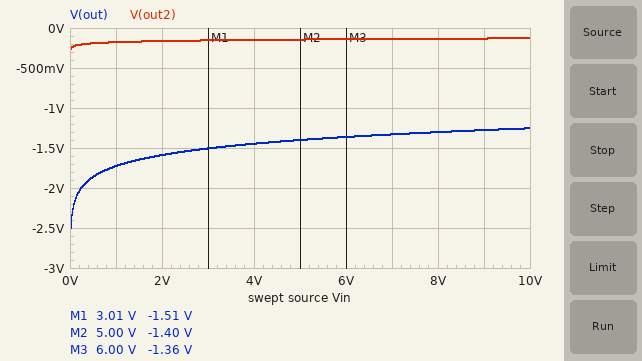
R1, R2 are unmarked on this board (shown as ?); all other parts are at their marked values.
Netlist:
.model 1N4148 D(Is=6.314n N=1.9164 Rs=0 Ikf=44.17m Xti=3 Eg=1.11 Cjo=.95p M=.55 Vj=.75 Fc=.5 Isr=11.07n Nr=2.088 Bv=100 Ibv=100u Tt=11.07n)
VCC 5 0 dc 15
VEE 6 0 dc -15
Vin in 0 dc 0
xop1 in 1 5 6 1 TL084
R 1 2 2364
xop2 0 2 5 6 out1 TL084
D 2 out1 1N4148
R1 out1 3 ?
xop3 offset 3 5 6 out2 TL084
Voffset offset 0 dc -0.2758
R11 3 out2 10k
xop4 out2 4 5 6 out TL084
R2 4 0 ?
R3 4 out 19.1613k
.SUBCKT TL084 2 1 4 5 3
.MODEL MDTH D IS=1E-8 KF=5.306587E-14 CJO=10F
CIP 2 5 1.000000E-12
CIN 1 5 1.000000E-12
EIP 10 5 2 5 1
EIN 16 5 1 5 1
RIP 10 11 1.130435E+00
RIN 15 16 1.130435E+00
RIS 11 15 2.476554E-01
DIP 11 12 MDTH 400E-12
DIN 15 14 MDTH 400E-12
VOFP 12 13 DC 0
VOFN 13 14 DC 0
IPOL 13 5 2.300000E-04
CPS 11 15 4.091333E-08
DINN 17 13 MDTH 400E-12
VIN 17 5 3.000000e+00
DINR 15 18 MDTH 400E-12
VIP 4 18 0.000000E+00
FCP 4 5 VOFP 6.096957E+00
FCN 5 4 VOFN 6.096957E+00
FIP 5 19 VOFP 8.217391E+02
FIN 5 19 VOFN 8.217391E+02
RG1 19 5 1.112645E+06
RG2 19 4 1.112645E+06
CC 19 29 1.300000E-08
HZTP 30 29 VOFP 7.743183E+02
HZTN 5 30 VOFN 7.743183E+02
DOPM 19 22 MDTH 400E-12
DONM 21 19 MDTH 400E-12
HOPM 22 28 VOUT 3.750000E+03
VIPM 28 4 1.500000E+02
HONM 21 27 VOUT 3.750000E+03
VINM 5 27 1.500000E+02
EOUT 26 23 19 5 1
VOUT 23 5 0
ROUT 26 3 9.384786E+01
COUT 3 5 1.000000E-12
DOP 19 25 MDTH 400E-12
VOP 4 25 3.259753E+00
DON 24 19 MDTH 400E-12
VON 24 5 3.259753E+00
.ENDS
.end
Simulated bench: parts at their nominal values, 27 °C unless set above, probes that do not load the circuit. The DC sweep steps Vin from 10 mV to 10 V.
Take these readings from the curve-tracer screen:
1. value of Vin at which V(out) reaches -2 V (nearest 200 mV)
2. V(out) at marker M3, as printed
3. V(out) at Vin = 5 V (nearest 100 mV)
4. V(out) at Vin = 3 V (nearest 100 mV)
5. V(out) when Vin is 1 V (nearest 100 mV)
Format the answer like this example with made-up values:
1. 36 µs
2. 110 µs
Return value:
1. 200 mV
2. -1.36 V
3. -1.4 V
4. -1.5 V
5. -1.7 V
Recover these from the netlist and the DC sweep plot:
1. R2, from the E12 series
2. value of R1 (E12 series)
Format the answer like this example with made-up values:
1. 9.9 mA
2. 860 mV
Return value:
1. 2.2 kΩ
2. 27 kΩ
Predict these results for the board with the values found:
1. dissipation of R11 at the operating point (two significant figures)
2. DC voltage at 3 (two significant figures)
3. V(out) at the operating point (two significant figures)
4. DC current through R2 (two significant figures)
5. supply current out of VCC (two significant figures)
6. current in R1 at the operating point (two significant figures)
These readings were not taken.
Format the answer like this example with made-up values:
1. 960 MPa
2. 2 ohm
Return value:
1. 1.0 µW
2. -280 mV
3. -3.7 V
4. 170 µA
5. 5.7 mA
6. 10 µA
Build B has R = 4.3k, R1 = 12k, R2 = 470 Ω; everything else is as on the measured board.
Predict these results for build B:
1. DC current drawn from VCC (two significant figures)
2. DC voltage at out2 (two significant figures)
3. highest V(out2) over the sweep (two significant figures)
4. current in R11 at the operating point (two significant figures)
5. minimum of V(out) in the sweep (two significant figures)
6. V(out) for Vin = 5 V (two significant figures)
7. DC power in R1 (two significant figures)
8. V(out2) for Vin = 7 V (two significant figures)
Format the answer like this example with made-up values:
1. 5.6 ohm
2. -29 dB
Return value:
1. 5.7 mA
2. -510 mV
3. 25 mV
4. 23 µA
5. -12 V
6. -350 mV
7. 6.3 µW
8. 7.6 mV
